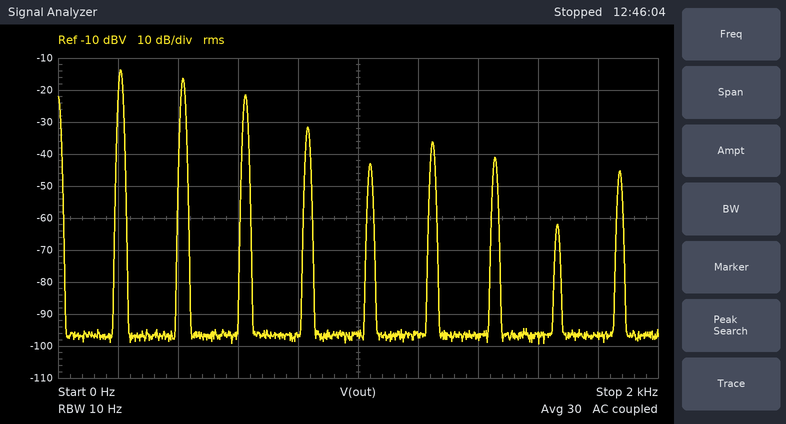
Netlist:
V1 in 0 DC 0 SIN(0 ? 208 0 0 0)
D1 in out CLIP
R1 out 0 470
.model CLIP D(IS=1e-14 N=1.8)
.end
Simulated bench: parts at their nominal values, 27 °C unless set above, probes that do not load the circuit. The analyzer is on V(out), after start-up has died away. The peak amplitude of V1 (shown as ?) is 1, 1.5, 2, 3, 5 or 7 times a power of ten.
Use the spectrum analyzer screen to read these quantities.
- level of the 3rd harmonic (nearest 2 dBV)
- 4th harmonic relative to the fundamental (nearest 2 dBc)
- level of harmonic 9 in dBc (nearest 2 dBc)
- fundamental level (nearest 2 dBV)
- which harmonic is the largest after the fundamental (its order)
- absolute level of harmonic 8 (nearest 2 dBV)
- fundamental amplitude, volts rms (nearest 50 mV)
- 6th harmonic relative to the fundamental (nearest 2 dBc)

-22 dBV
-18 dBc
-32 dBc
-14 dBV
2
-62 dBV
200 mV
-22 dBc
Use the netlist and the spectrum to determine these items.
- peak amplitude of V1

2 V
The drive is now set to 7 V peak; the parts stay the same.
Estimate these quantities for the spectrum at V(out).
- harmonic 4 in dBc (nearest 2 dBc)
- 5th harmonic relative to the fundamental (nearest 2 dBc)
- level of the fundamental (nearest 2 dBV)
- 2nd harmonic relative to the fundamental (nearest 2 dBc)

-22 dBc
-26 dBc
6 dBV
-6 dBc
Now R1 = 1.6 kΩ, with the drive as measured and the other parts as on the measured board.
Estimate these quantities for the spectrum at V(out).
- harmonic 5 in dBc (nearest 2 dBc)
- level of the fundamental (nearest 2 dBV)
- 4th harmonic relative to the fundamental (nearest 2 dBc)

-26 dBc
-12 dBV
-20 dBc
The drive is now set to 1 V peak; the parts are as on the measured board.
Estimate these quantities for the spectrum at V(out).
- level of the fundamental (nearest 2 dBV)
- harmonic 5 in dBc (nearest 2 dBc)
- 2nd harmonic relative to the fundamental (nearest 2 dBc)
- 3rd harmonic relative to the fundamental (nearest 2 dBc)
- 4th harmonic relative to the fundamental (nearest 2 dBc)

-60 dBV
-6 dBc
0 dBc
-2 dBc
-4 dBc
